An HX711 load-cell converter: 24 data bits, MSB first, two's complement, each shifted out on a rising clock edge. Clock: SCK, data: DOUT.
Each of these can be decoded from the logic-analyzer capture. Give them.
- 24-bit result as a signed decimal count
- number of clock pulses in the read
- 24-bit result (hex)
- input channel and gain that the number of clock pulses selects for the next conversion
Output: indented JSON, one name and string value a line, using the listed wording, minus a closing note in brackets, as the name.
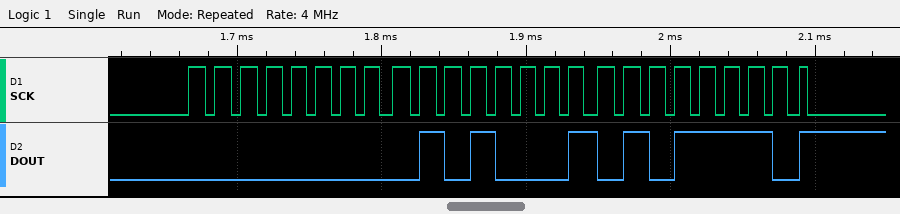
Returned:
{
  "24-bit result as a signed decimal count": "20830",
  "number of clock pulses in the read": "25",
  "24-bit result": "0x00515E",
  "input channel and gain that the number of clock pulses selects for the next conversion": "channel A, gain 128"
}
